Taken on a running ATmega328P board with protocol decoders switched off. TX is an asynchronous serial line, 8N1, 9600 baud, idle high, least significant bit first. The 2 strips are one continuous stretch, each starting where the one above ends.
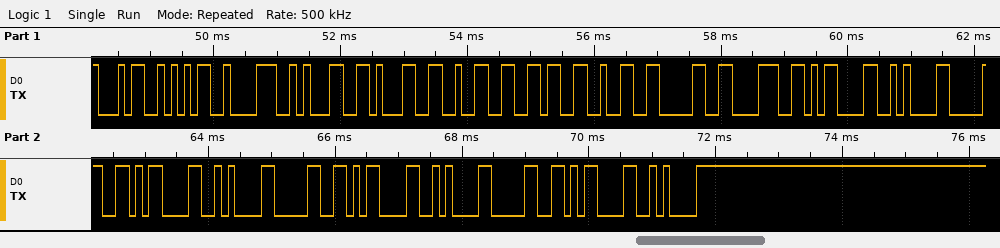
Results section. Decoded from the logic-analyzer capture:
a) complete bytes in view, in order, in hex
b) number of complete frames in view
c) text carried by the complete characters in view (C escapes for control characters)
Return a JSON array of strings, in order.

["0x34 0x35 0x38 0x31 0x31 0x32 0x36 0x32 0x30 0x38 0x0D 0x0A 0x30 0x0D 0x0A 0x30 0x0D 0x0A 0x30 0x0D 0x0A", "21", "\"4581126208\\r\\n0\\r\\n0\\r\\n0\\r\\n\""]
